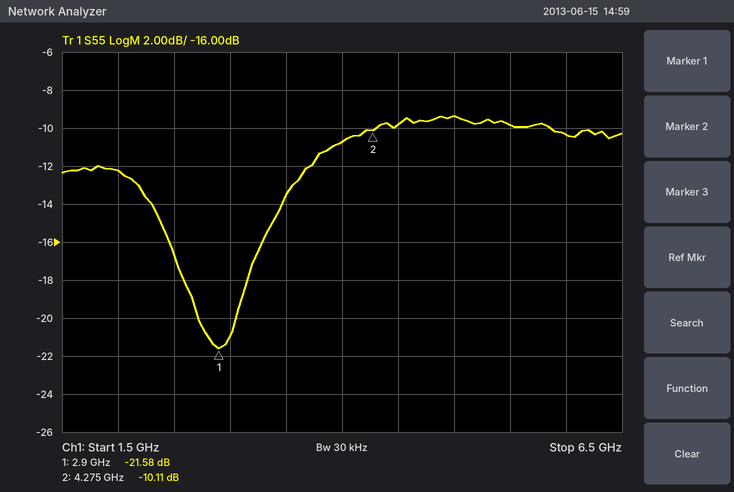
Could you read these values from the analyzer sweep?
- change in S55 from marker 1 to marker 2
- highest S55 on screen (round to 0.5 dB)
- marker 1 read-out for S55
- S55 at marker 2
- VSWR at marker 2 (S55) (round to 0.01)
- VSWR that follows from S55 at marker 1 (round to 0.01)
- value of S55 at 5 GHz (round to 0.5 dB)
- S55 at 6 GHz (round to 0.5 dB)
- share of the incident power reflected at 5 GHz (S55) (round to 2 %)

11.47 dB
-9.5 dB
-21.58 dB
-10.11 dB
1.91
1.18
-9.5 dB
-10.5 dB
12 %
